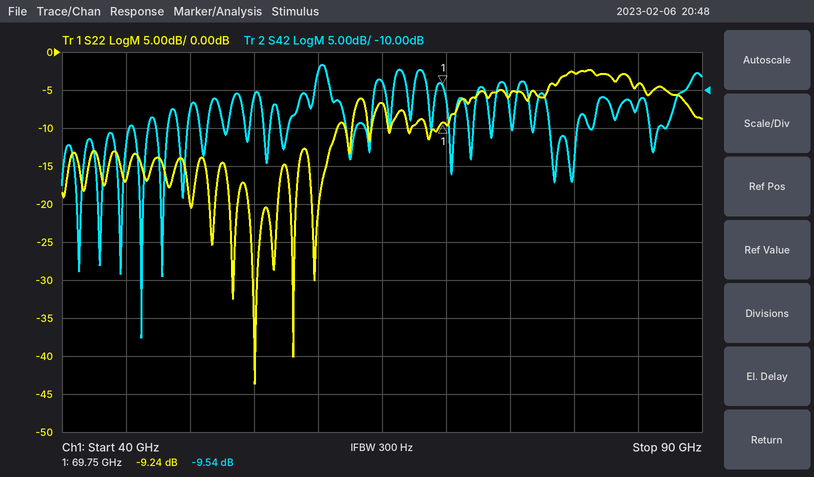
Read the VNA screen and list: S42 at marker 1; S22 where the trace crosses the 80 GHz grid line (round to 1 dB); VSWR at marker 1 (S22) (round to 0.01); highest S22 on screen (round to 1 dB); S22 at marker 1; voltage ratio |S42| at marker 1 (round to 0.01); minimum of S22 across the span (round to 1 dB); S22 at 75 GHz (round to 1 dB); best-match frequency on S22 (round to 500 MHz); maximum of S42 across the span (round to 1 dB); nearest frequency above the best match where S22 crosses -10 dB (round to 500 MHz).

-9.54 dB
-3 dB
2.05
-2 dB
-9.24 dB
0.33
-44 dB
-6 dB
55.0 GHz
-7 dB
61.5 GHz
